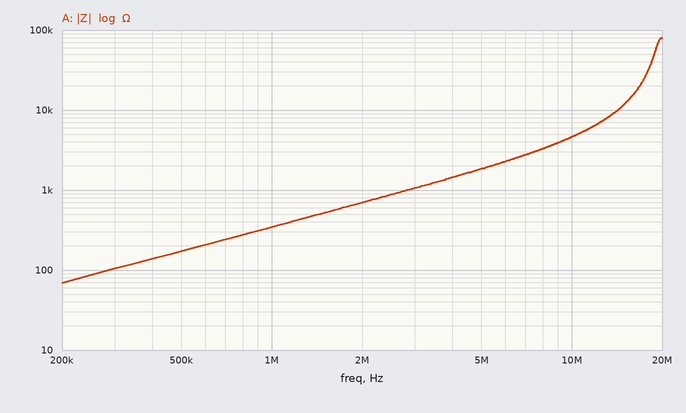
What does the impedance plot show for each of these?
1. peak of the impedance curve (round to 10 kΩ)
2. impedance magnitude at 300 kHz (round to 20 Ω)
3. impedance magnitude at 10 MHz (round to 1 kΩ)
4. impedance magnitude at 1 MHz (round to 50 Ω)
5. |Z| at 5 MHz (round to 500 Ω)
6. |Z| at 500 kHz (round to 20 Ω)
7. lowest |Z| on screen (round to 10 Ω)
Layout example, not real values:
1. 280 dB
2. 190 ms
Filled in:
1. 80 kΩ
2. 100 Ω
3. 5 kΩ
4. 350 Ω
5. 2.0 kΩ
6. 180 Ω
7. 70 Ω
